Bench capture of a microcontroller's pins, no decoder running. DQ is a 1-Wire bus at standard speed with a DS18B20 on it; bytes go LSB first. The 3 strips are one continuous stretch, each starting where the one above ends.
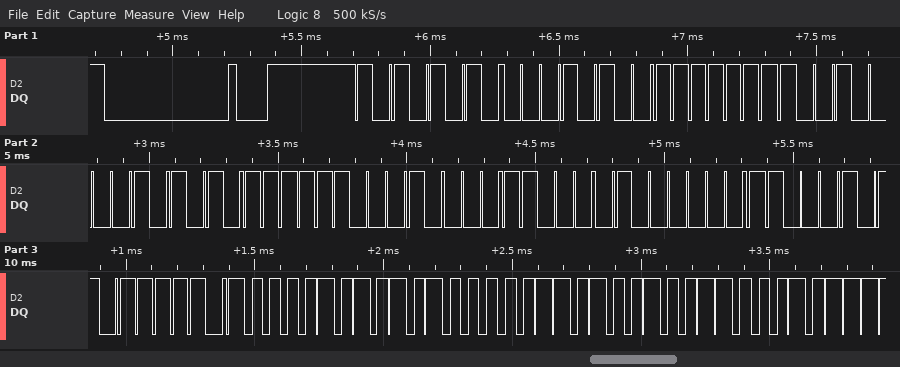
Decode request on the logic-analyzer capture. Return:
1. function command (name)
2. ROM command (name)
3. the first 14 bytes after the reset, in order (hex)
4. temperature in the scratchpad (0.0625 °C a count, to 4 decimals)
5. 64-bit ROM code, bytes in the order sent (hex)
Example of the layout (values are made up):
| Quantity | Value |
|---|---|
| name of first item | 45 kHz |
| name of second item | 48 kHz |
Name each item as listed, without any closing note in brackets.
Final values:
| Quantity | Value |
|---|---|
| function command | Read Scratchpad |
| ROM command | Match ROM |
| the first 14 bytes after the reset, in order | 55 28 FF 84 EA 47 18 02 A3 BE 50 05 4B 46 |
| temperature in the scratchpad | 85.0000 °C |
| 64-bit ROM code, bytes in the order sent | 28 FF 84 EA 47 18 02 A3 |
